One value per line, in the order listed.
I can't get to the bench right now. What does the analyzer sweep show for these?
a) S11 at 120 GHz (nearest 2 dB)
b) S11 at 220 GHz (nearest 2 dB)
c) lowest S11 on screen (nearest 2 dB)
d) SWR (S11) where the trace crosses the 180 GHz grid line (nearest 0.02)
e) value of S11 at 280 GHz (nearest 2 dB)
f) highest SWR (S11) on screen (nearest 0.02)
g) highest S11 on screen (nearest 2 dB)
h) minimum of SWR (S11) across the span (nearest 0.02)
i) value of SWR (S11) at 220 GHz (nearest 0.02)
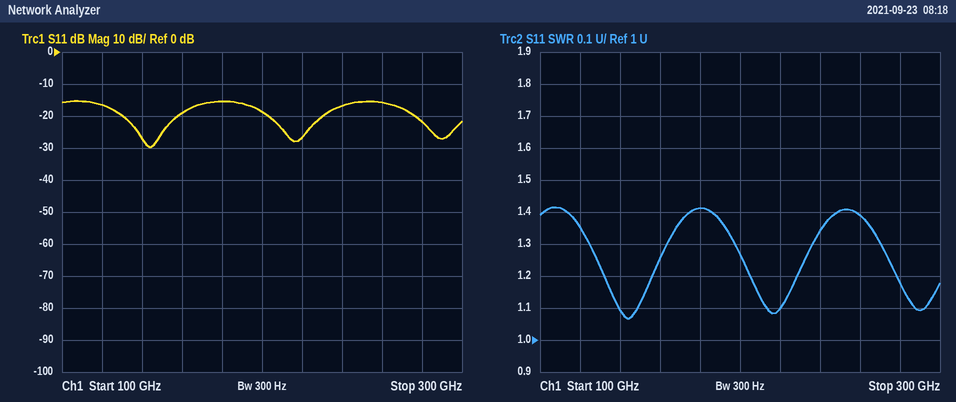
-16 dB
-26 dB
-30 dB
1.42
-22 dB
1.42
-16 dB
1.06
1.10
